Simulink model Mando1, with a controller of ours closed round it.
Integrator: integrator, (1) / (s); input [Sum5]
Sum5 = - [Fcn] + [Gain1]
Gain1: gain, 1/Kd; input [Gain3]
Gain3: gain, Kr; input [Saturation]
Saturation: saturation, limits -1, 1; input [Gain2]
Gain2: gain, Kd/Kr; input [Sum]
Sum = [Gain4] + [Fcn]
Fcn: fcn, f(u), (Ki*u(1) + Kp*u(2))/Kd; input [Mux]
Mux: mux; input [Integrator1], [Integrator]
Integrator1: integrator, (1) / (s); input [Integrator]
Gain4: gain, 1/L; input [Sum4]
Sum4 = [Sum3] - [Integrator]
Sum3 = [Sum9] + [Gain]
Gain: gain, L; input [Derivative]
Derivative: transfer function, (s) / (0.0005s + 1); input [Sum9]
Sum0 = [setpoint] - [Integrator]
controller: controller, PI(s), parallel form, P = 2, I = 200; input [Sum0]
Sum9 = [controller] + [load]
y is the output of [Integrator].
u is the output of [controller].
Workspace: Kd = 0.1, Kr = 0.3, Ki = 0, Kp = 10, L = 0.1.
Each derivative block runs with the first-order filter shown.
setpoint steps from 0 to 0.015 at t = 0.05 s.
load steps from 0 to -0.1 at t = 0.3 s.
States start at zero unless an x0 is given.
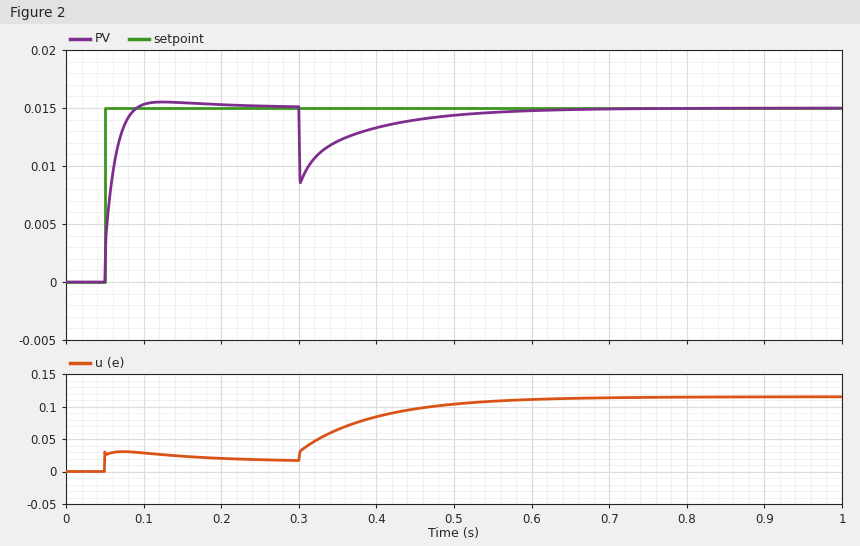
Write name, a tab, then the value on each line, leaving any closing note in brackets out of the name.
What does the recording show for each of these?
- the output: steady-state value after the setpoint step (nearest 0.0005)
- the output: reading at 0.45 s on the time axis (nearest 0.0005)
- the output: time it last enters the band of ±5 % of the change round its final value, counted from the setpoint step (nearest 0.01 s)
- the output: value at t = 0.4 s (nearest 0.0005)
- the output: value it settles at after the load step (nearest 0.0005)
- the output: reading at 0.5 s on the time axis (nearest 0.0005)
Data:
the output: steady-state value after the setpoint step	0.0150
the output: reading at 0.45 s on the time axis	0.0140
the output: time it last enters the band of ±5 % of the change round its final value, counted from the setpoint step	0.03 s
the output: value at t = 0.4 s	0.0135
the output: value it settles at after the load step	0.0150
the output: reading at 0.5 s on the time axis	0.0145
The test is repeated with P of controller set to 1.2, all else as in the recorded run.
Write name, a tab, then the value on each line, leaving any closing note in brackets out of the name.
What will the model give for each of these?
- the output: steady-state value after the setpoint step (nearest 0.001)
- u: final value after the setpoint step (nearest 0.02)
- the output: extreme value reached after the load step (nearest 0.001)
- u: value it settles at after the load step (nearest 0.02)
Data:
the output: steady-state value after the setpoint step	0.015
u: final value after the setpoint step	0.02
the output: extreme value reached after the load step	0.008
u: value it settles at after the load step	0.12
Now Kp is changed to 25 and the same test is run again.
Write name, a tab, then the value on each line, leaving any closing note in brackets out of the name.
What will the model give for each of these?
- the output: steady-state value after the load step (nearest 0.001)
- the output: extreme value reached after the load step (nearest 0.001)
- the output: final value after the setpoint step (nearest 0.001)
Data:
the output: steady-state value after the load step	0.012
the output: extreme value reached after the load step	0.005
the output: final value after the setpoint step	0.012
